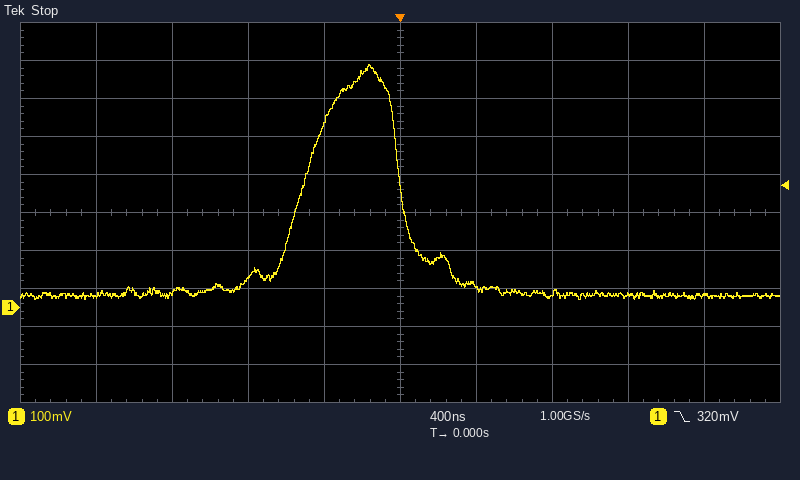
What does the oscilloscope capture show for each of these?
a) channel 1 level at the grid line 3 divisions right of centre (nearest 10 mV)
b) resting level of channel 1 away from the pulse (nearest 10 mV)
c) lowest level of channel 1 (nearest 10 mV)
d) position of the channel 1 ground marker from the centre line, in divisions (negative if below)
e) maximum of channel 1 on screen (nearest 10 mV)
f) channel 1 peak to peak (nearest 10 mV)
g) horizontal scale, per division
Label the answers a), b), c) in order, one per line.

a) 30 mV
b) 30 mV
c) 20 mV
d) -2.5 div
e) 640 mV
f) 620 mV
g) 400 ns
